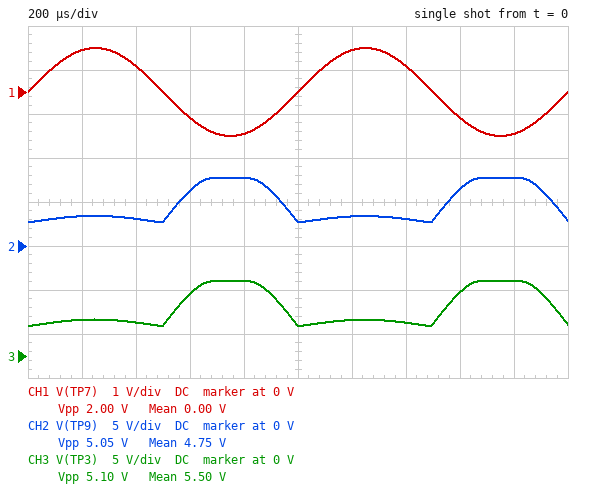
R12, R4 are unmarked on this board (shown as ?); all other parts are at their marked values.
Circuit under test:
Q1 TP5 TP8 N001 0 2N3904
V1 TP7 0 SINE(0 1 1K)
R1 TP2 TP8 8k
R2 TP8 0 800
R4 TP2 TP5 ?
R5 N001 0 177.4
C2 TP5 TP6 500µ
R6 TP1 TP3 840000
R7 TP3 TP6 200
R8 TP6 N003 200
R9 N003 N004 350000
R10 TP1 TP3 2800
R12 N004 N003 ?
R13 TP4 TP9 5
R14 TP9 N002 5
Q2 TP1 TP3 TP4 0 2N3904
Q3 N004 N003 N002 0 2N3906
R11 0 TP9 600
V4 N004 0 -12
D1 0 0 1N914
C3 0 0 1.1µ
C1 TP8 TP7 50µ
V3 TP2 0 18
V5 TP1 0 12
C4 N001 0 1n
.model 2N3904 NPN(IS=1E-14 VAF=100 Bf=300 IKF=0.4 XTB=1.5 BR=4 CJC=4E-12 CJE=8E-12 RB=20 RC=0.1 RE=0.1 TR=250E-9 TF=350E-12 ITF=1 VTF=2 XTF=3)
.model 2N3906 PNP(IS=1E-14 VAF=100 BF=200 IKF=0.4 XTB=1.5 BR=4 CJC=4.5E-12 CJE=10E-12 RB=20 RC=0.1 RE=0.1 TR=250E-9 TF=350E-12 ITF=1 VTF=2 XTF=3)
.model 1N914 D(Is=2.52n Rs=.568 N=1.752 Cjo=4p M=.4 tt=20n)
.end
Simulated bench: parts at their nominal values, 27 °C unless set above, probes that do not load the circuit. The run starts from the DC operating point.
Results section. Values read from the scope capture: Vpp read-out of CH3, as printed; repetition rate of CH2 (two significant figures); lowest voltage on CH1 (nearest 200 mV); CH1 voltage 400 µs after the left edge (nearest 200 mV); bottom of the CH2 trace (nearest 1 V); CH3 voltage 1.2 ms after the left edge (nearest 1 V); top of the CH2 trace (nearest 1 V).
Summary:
5.10 V
1.0 kHz
-1.0 V
600 mV
3 V
4 V
8 V
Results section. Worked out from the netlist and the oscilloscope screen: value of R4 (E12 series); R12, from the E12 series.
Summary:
3.9 kΩ
4.7 kΩ
